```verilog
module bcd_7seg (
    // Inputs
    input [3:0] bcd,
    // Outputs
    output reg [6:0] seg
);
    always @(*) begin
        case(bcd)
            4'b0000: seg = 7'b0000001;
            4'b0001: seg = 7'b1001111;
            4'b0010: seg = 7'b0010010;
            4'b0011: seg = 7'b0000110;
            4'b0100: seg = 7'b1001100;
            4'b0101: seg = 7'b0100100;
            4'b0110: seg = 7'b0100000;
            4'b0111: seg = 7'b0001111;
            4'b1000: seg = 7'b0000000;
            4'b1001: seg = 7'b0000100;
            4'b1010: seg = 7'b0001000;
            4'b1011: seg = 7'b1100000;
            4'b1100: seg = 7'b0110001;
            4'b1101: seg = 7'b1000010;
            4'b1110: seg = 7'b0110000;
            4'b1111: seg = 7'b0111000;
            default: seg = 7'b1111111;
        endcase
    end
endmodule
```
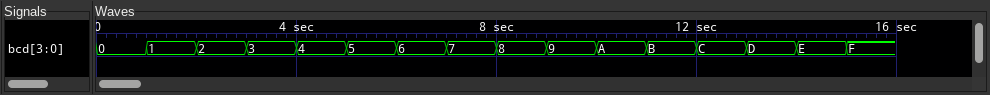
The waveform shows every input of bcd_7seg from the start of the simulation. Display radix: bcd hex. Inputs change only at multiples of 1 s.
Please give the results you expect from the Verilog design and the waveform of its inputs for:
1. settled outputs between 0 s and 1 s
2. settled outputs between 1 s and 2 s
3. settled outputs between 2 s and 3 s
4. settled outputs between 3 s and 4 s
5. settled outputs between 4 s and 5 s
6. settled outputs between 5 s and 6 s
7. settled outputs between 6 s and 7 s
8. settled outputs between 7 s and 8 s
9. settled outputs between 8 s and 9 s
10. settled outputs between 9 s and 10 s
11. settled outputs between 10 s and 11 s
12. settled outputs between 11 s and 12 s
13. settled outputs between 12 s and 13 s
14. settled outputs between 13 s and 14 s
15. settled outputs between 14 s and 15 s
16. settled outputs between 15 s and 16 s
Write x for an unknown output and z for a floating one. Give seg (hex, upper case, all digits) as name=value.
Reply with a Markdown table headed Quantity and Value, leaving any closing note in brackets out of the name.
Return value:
| Quantity | Value |
|---|---|
| settled outputs between 0 s and 1 s | seg=01 |
| settled outputs between 1 s and 2 s | seg=4F |
| settled outputs between 2 s and 3 s | seg=12 |
| settled outputs between 3 s and 4 s | seg=06 |
| settled outputs between 4 s and 5 s | seg=4C |
| settled outputs between 5 s and 6 s | seg=24 |
| settled outputs between 6 s and 7 s | seg=20 |
| settled outputs between 7 s and 8 s | seg=0F |
| settled outputs between 8 s and 9 s | seg=00 |
| settled outputs between 9 s and 10 s | seg=04 |
| settled outputs between 10 s and 11 s | seg=08 |
| settled outputs between 11 s and 12 s | seg=60 |
| settled outputs between 12 s and 13 s | seg=31 |
| settled outputs between 13 s and 14 s | seg=42 |
| settled outputs between 14 s and 15 s | seg=30 |
| settled outputs between 15 s and 16 s | seg=38 |
